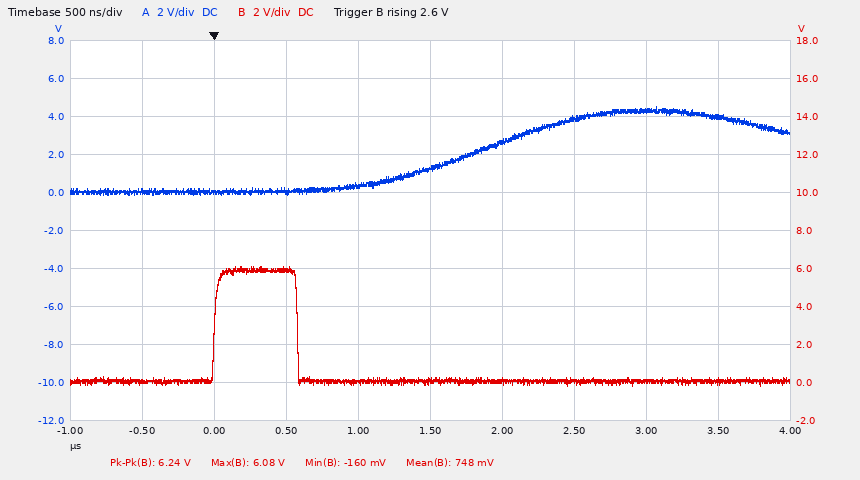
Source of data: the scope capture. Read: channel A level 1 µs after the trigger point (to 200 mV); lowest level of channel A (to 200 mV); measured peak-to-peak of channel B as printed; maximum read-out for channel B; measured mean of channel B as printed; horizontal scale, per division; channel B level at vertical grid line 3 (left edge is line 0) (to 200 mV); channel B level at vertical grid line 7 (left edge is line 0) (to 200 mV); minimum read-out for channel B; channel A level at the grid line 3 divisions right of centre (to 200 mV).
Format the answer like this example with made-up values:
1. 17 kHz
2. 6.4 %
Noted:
1. 400 mV
2. -200 mV
3. 6.24 V
4. 6.08 V
5. 748 mV
6. 500 ns
7. 6.0 V
8. 0.0 V
9. -160 mV
10. 4.4 V
